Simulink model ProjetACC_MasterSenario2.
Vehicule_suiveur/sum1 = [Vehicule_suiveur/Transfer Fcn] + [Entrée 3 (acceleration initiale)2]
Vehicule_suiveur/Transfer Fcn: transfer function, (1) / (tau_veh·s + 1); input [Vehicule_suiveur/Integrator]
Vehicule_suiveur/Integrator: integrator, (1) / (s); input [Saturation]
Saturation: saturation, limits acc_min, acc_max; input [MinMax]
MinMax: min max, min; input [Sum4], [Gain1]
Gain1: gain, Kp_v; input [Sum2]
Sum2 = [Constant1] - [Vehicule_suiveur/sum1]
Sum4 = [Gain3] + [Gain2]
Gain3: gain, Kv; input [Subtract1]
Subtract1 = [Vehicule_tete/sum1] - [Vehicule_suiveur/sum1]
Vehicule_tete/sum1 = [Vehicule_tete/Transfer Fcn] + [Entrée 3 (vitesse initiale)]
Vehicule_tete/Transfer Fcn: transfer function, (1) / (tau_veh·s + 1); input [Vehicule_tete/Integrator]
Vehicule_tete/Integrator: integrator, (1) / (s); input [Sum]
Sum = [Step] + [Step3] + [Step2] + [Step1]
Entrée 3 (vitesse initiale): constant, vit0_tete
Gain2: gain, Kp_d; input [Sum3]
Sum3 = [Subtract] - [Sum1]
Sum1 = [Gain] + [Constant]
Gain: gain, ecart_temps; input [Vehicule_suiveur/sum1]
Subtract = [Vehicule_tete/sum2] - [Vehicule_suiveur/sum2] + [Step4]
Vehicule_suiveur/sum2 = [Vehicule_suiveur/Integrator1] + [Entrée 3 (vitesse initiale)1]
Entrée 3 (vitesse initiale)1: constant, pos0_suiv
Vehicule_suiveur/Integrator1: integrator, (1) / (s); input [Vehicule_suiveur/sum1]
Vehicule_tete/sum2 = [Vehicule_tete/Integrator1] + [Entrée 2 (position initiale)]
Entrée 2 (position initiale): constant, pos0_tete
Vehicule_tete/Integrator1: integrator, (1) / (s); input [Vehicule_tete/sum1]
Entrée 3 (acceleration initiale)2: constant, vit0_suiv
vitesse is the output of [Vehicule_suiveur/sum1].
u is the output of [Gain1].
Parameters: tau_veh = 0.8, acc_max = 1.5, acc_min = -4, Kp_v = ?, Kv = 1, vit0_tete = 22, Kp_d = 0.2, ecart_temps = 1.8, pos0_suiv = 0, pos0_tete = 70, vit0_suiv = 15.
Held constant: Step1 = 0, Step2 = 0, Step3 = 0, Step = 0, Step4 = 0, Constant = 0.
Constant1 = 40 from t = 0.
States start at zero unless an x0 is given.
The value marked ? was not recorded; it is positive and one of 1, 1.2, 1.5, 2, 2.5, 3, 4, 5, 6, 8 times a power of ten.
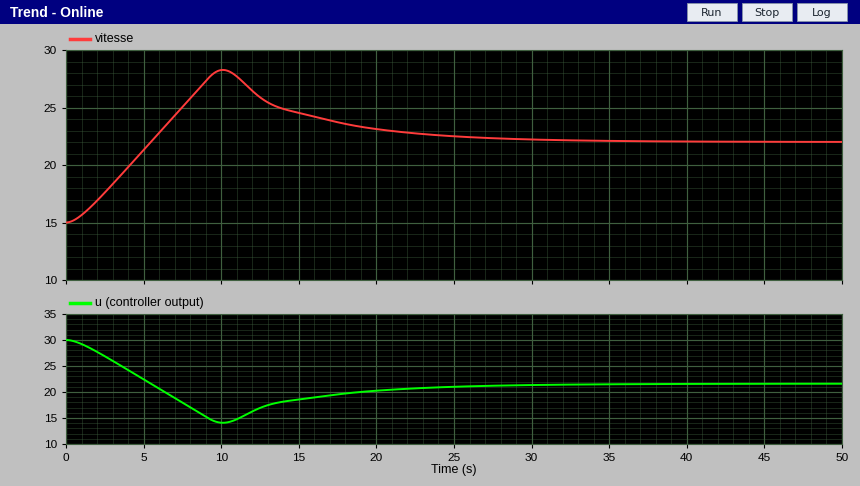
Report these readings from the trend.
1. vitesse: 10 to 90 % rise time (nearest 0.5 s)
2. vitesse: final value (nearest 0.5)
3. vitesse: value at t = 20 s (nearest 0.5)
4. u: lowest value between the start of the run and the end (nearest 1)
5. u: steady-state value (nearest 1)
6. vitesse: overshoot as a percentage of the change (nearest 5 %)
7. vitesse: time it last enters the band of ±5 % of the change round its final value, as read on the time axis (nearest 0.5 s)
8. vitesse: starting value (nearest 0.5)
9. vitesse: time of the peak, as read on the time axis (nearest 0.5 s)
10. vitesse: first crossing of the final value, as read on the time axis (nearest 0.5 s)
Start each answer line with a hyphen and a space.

- 4.0 s
- 22.0
- 23.0
- 14
- 22
- 90 %
- 27.0 s
- 15.0
- 10.0 s
- 5.5 s
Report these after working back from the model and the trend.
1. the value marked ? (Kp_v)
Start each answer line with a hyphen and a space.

- 1.2
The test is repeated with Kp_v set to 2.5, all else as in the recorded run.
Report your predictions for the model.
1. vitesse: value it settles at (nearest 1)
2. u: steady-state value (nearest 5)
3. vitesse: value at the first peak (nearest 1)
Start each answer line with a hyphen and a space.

- 22
- 45
- 28
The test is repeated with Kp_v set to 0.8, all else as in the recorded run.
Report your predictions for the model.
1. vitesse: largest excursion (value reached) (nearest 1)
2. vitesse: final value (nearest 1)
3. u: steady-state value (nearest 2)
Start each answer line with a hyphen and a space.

- 28
- 22
- 14
